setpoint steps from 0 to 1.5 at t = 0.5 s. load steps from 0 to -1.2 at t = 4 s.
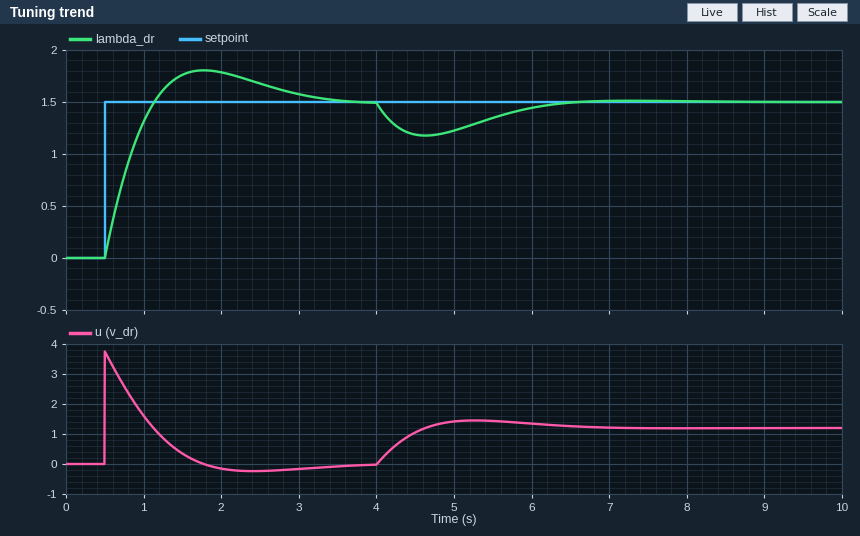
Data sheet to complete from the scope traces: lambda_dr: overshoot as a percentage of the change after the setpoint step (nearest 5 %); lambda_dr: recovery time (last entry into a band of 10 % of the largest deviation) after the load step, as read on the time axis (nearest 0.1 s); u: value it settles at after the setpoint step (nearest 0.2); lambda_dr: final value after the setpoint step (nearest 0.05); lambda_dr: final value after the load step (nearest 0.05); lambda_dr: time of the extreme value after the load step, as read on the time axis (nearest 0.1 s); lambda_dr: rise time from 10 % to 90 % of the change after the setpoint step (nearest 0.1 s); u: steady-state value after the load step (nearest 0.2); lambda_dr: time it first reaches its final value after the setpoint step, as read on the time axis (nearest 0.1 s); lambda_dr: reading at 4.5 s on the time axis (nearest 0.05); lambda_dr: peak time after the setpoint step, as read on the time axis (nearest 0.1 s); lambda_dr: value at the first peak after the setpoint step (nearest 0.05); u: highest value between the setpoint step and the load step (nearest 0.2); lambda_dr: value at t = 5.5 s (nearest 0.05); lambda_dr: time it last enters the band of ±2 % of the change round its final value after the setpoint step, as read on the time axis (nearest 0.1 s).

20 %
6.2 s
0.0
1.50
1.50
4.6 s
0.5 s
1.2
1.1 s
1.20
1.8 s
1.80
3.8
1.35
3.3 s
